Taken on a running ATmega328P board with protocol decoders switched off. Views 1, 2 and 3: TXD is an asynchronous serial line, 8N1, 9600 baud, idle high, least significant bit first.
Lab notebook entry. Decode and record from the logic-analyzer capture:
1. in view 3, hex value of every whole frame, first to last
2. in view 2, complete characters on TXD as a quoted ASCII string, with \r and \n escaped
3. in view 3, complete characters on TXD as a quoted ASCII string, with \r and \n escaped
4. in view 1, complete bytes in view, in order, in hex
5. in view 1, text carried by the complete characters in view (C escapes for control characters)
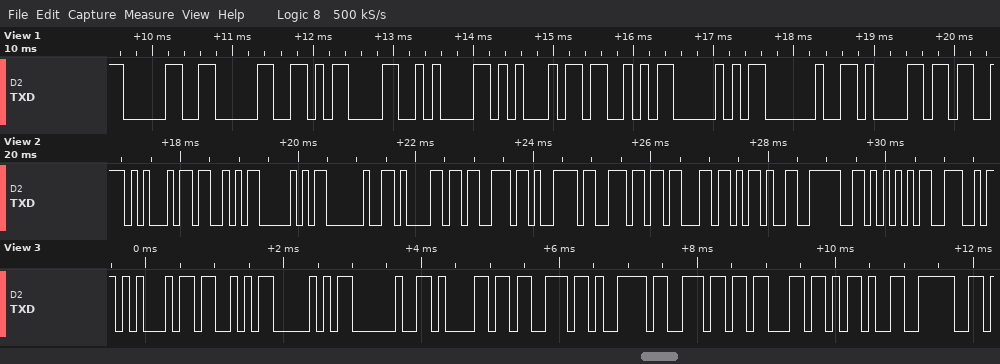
45 53 50 20 61 73 79 6E 63 2D 3E
"ESP async->UN"
"ESP async->"
30 30 0D 0A 45 53 50 20 61
"00\r\nESP a"
